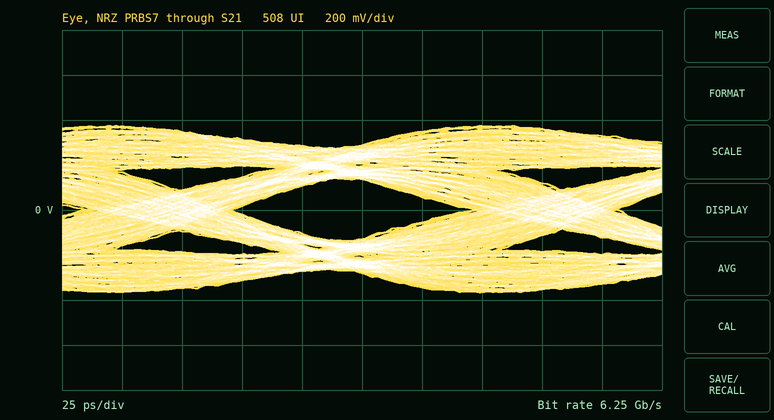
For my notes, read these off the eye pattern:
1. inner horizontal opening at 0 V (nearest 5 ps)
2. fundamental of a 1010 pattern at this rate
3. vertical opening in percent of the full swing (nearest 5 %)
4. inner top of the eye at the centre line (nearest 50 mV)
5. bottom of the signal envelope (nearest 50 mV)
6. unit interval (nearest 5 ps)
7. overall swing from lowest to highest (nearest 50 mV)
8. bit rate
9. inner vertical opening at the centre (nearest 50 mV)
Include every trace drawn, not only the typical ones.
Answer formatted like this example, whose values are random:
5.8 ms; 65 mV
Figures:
100 ps; 3.125 GHz; 35 %; 150 mV; -350 mV; 160 ps; 750 mV; 6.25 Gb/s; 250 mV
